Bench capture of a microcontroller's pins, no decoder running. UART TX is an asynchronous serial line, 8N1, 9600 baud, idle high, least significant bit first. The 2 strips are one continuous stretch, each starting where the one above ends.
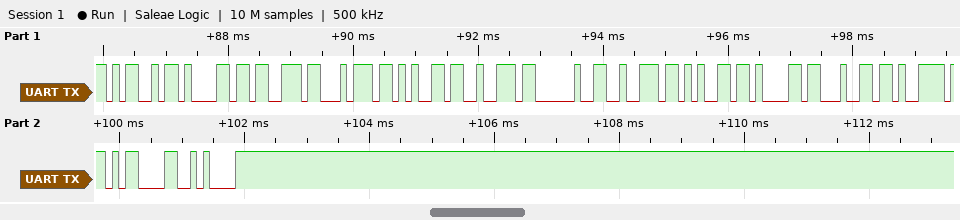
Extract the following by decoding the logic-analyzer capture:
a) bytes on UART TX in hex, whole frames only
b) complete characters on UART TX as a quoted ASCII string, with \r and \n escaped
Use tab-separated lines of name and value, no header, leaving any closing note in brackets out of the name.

bytes on UART TX in hex, whole frames only	4D 61 73 74 65 72 20 72 65 61 64 79 0D 0A
complete characters on UART TX as a quoted ASCII string, with \r and \n escaped	"Master ready\r\n"
